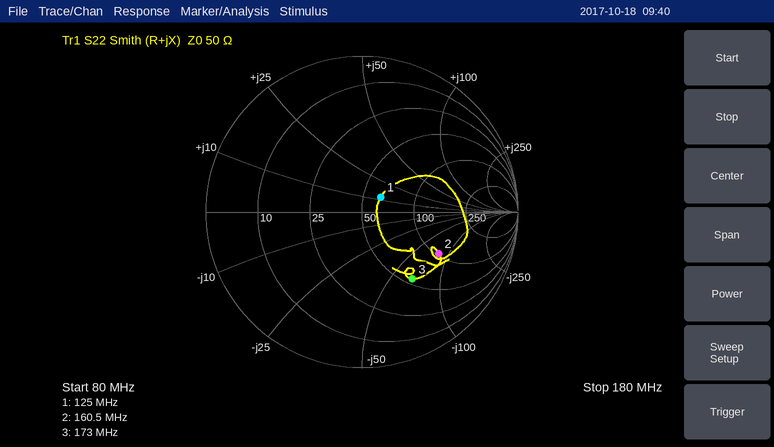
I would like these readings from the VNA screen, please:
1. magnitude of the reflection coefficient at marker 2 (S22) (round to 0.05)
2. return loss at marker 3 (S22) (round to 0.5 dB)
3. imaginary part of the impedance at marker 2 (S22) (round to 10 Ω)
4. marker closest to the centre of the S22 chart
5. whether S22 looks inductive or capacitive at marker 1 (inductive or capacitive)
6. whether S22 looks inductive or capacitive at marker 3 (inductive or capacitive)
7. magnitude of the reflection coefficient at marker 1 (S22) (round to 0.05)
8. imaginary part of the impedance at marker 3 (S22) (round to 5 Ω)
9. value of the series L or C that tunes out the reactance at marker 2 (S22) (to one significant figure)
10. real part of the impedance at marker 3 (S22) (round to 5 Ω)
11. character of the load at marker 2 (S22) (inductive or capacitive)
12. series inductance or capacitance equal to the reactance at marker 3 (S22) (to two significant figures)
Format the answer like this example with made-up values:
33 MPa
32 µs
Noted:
0.55
5.5 dB
-80 Ω
marker 1
inductive
capacitive
0.15
-65 Ω
80 nH
55 Ω
capacitive
14 pF
